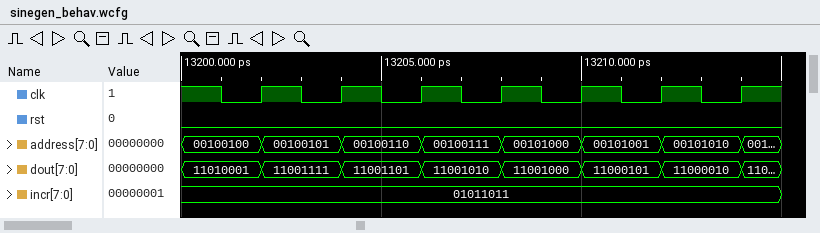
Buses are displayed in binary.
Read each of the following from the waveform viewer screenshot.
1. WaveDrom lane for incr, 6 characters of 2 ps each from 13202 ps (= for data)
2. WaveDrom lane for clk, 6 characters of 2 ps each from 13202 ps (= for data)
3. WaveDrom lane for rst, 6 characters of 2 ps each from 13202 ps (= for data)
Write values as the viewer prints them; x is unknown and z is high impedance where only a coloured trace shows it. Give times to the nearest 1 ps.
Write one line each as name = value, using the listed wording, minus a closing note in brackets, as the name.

WaveDrom lane for incr, 6 characters of 2 ps each from 13202 ps = {name: 'incr', wave: '=.....', data: '01011011'}
WaveDrom lane for clk, 6 characters of 2 ps each from 13202 ps = {name: 'clk', wave: 'p.....'}
WaveDrom lane for rst, 6 characters of 2 ps each from 13202 ps = {name: 'rst', wave: '0.....'}
